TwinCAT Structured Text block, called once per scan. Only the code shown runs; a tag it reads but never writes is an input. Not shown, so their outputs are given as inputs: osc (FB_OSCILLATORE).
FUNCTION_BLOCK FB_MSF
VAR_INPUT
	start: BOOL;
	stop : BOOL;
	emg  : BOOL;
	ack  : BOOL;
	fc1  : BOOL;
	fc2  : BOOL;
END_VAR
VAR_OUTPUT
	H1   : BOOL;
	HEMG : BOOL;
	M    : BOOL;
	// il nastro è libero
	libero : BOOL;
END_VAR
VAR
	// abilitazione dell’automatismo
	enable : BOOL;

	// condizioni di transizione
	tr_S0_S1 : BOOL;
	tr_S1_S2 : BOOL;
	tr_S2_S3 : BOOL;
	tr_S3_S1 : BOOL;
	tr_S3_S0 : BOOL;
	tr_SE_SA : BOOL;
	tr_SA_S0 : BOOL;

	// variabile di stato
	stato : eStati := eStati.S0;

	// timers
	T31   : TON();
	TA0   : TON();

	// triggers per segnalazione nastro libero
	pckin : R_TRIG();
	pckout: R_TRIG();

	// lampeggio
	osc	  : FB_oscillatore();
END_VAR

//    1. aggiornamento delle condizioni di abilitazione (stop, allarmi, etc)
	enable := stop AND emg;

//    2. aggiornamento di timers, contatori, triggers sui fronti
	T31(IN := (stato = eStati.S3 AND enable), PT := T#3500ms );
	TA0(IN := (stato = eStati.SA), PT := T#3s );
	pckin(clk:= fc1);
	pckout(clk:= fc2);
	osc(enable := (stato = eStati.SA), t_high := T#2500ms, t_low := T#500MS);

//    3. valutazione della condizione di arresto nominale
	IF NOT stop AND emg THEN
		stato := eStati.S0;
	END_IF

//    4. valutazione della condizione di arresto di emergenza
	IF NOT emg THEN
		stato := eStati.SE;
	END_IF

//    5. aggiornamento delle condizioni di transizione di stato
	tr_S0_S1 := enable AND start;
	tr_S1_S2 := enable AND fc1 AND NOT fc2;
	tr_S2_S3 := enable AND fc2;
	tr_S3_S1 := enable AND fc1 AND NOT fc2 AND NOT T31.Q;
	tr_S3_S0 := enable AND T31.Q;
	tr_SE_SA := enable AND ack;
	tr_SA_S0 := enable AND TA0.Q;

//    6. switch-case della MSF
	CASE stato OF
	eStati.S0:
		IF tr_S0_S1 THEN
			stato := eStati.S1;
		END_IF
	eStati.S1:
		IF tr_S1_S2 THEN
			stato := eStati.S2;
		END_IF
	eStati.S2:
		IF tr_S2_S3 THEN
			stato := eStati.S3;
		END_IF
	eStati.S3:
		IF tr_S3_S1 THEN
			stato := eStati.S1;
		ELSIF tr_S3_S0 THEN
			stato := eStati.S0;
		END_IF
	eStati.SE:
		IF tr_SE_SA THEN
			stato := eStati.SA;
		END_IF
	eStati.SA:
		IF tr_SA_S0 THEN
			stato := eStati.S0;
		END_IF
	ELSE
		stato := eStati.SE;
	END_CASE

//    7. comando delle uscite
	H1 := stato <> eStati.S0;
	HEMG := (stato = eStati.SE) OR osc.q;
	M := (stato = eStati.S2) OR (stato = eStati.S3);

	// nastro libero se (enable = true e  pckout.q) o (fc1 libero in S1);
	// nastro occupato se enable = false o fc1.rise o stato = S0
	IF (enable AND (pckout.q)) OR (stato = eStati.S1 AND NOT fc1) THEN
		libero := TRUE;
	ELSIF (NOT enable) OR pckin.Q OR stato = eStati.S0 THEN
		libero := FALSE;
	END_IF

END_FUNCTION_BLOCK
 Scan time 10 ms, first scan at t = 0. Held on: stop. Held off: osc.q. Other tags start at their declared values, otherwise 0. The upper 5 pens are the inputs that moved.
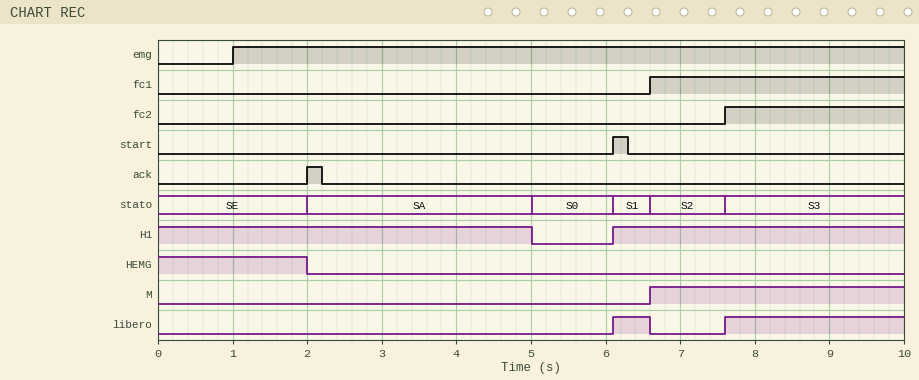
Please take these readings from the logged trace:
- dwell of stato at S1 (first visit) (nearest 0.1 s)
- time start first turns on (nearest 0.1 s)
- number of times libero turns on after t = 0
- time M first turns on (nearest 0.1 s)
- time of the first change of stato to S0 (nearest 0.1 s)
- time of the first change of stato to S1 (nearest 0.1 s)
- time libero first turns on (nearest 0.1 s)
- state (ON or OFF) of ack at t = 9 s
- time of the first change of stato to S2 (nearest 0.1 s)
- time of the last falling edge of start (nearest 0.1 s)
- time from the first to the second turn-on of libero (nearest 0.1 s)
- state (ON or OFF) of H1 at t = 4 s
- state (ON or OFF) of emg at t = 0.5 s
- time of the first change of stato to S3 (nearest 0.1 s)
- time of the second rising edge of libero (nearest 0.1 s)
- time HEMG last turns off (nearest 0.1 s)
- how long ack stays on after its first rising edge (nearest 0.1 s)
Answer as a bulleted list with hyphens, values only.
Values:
- 0.5 s
- 6.1 s
- 2
- 6.6 s
- 5.0 s
- 6.1 s
- 6.1 s
- OFF
- 6.6 s
- 6.3 s
- 1.5 s
- ON
- OFF
- 7.6 s
- 7.6 s
- 2.0 s
- 0.2 s
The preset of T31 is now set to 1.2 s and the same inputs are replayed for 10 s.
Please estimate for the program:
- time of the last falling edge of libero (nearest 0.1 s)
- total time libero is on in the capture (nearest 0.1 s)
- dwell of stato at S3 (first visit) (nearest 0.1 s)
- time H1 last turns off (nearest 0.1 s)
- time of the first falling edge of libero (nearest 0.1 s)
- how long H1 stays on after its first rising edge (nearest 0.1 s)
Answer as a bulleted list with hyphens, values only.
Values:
- 8.8 s
- 1.7 s
- 1.2 s
- 8.8 s
- 6.6 s
- 2.7 s
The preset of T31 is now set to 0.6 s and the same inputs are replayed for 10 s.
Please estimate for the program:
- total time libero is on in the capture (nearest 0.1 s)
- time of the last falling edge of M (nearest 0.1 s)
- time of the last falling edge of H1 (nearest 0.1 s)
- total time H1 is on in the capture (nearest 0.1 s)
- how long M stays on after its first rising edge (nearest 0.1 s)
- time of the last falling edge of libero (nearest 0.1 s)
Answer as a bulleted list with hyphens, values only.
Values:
- 1.1 s
- 8.2 s
- 8.2 s
- 7.1 s
- 1.6 s
- 8.2 s
